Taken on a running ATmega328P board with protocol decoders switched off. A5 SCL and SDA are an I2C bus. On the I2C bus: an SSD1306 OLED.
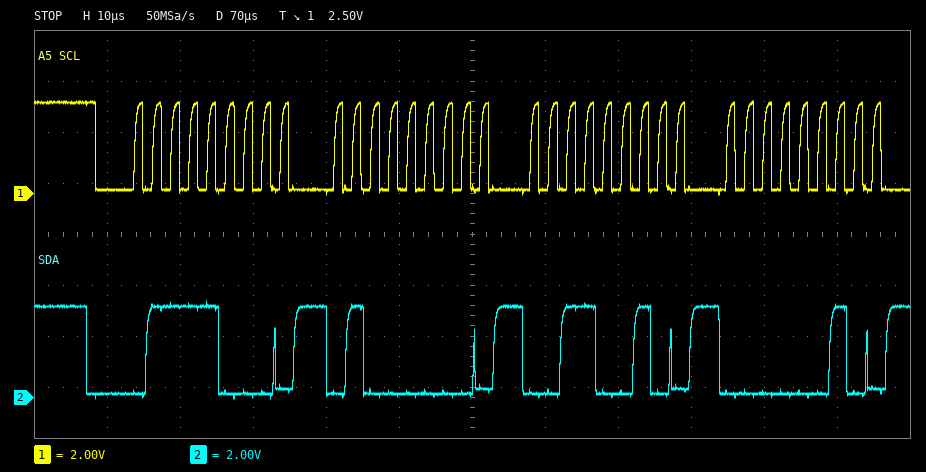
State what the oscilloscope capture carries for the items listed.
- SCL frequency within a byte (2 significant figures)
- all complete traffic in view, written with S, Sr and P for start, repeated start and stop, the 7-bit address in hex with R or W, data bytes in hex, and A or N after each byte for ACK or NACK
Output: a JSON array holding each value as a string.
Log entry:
["400 kHz", "S 3CW A 40 A 32 A 02 A"]
